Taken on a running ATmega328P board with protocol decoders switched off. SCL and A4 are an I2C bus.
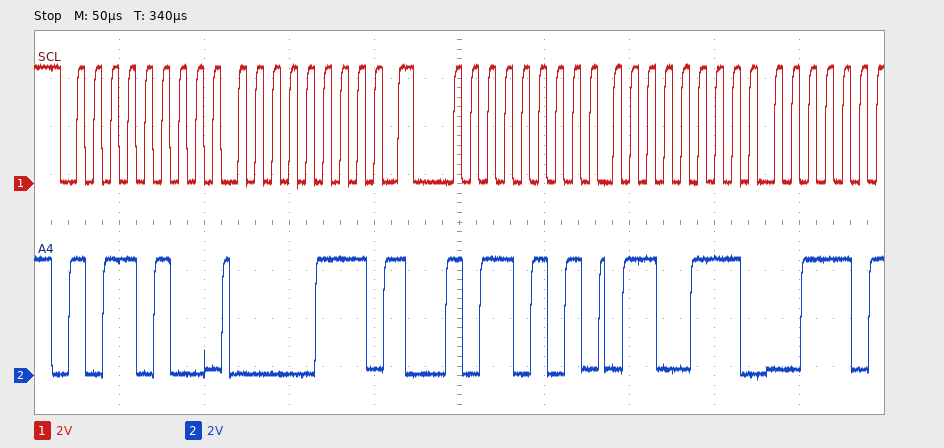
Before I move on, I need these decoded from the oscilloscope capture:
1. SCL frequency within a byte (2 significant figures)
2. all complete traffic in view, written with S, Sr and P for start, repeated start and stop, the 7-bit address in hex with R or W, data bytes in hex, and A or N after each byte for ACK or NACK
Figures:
100 kHz
S 5AW A 07 A Sr 5AR A 67 A
